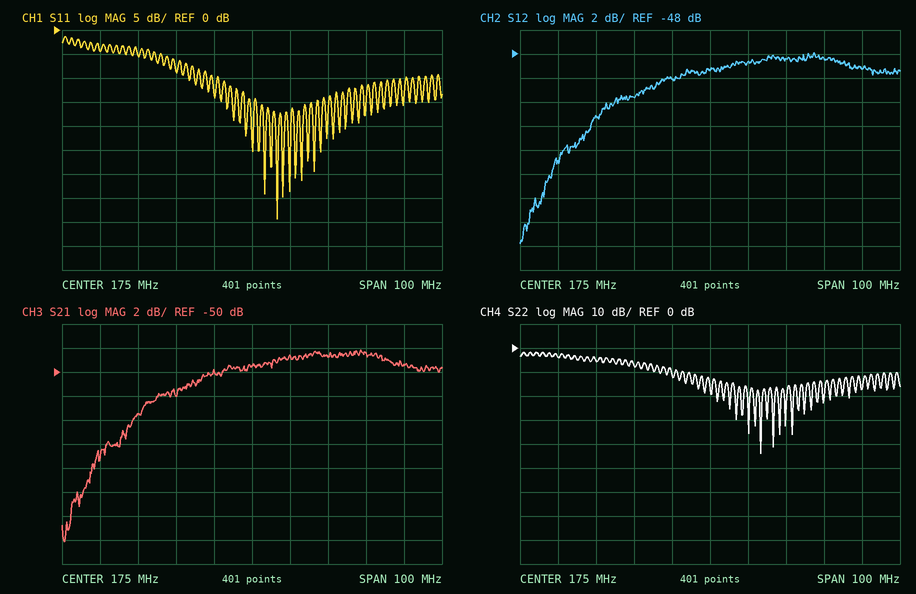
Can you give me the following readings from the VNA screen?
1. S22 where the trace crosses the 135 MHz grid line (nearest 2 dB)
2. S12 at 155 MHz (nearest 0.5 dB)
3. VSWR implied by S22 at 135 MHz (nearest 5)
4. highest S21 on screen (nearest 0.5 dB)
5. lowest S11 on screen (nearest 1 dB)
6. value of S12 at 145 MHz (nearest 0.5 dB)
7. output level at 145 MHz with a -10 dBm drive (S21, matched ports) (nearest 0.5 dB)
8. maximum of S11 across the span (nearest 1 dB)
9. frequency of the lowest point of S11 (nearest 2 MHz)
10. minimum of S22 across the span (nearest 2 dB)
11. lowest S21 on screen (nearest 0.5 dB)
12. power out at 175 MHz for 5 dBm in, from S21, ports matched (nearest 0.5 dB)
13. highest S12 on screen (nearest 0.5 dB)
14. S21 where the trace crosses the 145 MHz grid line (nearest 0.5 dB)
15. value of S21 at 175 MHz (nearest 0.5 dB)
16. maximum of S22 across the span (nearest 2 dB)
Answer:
-4 dB
-51.5 dB
5
-48.0 dB
-39 dB
-53.0 dB
-63.5 dBm
-1 dB
182 MHz
-44 dB
-64.0 dB
-44.5 dBm
-48.0 dB
-53.5 dB
-49.5 dB
-2 dB
